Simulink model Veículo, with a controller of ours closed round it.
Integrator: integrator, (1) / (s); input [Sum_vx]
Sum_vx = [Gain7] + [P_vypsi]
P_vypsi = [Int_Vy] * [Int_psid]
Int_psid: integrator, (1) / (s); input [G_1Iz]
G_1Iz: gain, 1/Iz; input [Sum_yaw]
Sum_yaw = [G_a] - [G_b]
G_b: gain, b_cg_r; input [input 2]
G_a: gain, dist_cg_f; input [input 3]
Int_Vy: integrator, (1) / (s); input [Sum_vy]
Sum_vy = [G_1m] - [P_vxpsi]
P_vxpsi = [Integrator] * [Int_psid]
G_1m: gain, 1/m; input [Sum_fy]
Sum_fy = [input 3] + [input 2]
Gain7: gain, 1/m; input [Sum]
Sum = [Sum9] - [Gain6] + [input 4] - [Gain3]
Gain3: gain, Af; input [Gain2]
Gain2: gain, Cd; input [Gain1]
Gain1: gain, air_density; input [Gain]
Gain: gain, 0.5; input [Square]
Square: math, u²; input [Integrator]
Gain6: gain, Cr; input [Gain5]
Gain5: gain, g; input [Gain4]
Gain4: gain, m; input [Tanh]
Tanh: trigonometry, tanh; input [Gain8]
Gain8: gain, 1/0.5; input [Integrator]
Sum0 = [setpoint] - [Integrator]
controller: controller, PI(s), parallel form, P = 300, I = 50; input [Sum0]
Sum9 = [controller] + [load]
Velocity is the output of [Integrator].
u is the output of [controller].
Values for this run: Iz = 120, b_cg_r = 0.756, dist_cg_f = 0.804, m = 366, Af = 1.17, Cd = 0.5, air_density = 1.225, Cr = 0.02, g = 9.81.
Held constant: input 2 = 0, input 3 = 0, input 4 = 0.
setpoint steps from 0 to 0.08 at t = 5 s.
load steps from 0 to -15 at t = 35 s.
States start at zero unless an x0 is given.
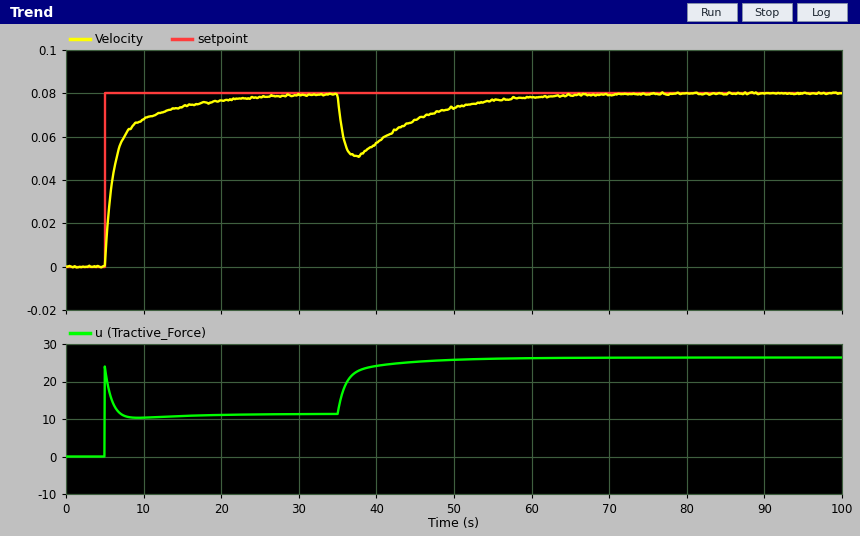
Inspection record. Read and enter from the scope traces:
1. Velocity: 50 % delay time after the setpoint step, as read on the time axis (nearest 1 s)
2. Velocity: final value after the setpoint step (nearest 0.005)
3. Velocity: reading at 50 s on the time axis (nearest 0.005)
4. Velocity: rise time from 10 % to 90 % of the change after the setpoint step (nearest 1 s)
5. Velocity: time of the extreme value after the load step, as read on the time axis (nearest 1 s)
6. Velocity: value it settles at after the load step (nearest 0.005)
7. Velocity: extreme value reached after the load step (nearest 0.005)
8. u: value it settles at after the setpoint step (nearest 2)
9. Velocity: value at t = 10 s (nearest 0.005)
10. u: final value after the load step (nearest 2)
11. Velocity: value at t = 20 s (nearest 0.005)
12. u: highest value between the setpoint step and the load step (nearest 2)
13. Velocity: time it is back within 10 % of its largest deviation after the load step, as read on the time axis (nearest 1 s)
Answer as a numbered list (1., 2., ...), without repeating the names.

1. 6 s
2. 0.080
3. 0.075
4. 8 s
5. 37 s
6. 0.080
7. 0.050
8. 12
9. 0.070
10. 26
11. 0.075
12. 24
13. 57 s
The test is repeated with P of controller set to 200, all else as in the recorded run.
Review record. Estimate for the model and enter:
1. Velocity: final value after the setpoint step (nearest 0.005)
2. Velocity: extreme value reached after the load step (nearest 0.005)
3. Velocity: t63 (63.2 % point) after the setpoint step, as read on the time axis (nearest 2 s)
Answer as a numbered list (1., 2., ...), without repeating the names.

1. 0.080
2. 0.045
3. 8 s
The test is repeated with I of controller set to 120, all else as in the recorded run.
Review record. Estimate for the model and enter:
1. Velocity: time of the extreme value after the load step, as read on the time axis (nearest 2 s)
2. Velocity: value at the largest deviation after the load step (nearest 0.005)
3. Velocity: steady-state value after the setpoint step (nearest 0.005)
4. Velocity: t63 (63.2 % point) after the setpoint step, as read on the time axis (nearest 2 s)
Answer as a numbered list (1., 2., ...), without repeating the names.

1. 36 s
2. 0.055
3. 0.080
4. 6 s
